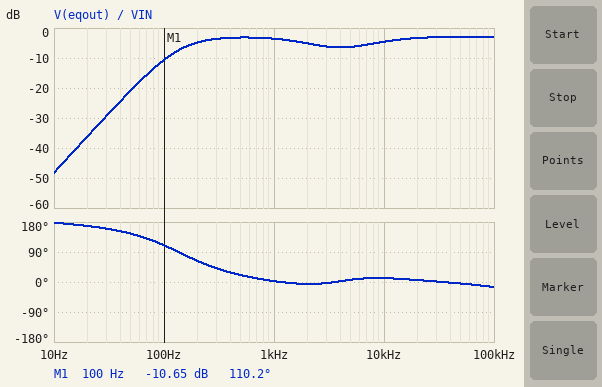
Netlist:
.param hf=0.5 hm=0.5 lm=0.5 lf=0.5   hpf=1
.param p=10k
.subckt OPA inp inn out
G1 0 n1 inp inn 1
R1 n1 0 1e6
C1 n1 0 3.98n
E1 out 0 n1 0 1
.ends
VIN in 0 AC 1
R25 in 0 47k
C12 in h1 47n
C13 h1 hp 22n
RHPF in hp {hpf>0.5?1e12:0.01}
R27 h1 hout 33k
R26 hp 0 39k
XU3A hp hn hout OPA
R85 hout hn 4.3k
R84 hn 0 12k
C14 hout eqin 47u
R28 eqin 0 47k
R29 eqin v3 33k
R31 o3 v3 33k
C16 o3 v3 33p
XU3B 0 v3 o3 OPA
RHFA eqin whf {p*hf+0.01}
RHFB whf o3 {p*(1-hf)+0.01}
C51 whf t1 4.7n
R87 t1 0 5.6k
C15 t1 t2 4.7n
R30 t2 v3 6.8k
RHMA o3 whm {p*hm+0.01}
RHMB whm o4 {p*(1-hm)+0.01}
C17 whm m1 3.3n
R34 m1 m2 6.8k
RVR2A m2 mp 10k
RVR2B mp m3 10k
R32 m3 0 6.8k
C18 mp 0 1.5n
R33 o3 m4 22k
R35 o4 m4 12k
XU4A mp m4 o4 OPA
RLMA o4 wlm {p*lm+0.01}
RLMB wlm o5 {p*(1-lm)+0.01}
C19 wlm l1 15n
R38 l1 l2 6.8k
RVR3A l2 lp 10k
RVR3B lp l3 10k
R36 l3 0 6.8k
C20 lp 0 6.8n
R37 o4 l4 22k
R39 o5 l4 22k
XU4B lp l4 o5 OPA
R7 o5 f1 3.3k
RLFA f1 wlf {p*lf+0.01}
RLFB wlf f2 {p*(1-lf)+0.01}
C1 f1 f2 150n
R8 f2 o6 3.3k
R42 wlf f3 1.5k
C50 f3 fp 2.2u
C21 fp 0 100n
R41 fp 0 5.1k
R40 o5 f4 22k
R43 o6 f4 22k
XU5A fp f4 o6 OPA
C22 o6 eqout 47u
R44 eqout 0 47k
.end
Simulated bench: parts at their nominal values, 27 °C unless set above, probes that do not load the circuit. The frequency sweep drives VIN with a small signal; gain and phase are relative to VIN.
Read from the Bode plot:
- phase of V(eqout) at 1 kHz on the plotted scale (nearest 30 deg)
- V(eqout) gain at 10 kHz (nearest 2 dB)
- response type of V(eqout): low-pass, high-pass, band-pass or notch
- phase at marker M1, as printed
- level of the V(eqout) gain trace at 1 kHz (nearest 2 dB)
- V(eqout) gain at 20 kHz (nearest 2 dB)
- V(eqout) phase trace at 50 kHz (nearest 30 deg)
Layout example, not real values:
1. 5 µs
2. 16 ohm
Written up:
1. 0 deg
2. -4 dB
3. high-pass
4. 110.2 deg
5. -4 dB
6. -4 dB
7. 0 deg
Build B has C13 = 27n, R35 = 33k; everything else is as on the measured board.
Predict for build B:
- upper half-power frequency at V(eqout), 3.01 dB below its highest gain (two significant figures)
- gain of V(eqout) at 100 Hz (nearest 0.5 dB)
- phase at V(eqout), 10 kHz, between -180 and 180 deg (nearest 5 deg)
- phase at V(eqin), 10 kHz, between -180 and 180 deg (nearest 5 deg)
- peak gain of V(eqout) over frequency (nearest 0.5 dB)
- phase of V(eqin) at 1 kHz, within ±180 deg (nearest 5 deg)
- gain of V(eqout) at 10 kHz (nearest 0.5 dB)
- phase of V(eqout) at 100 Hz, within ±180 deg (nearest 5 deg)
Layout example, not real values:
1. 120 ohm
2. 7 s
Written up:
1. 140 kHz
2. 0 dB
3. -10 deg
4. 0 deg
5. 8.5 dB
6. 10 deg
7. 7.0 dB
8. 105 deg
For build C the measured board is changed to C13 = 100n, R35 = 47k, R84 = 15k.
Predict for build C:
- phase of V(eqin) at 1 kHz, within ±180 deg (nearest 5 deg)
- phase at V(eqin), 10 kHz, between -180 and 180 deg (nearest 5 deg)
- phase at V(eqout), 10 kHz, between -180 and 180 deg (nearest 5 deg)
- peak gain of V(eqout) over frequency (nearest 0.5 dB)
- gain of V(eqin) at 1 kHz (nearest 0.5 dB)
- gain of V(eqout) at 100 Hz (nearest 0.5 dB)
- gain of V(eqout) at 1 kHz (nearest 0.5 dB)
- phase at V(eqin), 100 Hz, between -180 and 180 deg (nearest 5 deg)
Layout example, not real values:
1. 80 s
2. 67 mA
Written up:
1. 5 deg
2. 0 deg
3. -20 deg
4. 14.0 dB
5. 2.0 dB
6. 7.5 dB
7. 10.0 dB
8. 60 deg
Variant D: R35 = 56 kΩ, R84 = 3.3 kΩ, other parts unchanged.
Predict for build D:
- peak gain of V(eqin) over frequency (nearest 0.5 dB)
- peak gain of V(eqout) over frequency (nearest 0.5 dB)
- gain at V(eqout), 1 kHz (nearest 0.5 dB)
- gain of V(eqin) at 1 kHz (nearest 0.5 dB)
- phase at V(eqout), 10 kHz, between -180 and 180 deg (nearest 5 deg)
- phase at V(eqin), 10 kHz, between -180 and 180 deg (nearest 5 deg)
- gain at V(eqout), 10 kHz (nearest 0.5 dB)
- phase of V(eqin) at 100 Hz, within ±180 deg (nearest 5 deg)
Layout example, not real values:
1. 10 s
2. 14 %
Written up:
1. 8.5 dB
2. 22.5 dB
3. 17.0 dB
4. 7.5 dB
5. -25 deg
6. 0 deg
7. 18.0 dB
8. 125 deg
